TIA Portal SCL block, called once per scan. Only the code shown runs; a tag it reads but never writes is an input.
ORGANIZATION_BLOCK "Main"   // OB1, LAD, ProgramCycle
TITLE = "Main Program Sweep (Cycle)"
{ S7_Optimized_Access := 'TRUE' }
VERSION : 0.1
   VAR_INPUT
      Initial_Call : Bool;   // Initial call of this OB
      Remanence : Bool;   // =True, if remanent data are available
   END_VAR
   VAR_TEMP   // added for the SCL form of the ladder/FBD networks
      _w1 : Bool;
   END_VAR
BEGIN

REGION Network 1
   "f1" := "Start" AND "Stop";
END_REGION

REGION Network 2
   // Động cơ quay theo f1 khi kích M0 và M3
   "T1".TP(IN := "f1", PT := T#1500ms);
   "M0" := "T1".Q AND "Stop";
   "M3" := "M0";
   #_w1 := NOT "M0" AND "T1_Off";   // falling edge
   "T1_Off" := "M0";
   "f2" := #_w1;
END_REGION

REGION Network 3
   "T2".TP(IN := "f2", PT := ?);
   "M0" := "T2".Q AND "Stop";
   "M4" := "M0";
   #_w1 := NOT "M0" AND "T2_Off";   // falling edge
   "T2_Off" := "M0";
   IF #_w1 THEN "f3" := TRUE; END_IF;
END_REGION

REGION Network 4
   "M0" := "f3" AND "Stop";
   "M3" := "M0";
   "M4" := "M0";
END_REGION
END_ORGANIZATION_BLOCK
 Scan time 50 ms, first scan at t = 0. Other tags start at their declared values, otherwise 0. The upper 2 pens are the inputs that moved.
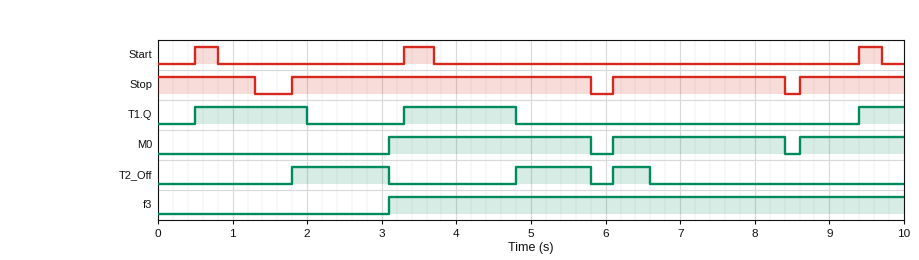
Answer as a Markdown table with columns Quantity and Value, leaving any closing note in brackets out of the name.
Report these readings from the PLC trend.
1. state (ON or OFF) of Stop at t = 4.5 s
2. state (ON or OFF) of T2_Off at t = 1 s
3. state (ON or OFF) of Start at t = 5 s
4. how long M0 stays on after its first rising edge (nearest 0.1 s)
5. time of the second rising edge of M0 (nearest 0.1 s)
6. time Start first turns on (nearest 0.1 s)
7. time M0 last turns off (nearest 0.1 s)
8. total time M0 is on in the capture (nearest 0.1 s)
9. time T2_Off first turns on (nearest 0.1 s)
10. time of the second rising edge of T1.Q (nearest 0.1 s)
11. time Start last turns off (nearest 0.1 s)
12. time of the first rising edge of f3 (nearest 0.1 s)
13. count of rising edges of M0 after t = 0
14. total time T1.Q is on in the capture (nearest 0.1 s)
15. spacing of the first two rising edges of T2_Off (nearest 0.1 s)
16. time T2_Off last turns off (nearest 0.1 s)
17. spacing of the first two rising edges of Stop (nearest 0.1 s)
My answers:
| Quantity | Value |
|---|---|
| state (ON or OFF) of Stop at t = 4.5 s | ON |
| state (ON or OFF) of T2_Off at t = 1 s | OFF |
| state (ON or OFF) of Start at t = 5 s | OFF |
| how long M0 stays on after its first rising edge | 2.7 s |
| time of the second rising edge of M0 | 6.1 s |
| time Start first turns on | 0.5 s |
| time M0 last turns off | 8.4 s |
| total time M0 is on in the capture | 6.4 s |
| time T2_Off first turns on | 1.8 s |
| time of the second rising edge of T1.Q | 3.3 s |
| time Start last turns off | 9.7 s |
| time of the first rising edge of f3 | 3.1 s |
| count of rising edges of M0 after t = 0 | 3 |
| total time T1.Q is on in the capture | 3.6 s |
| spacing of the first two rising edges of T2_Off | 3.0 s |
| time T2_Off last turns off | 6.6 s |
| spacing of the first two rising edges of Stop | 4.3 s |
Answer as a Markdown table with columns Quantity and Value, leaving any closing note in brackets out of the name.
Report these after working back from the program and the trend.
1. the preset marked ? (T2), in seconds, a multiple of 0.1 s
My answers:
| Quantity | Value |
|---|---|
| the preset marked ? (T2), in seconds, a multiple of 0.1 s | 1.8 s |
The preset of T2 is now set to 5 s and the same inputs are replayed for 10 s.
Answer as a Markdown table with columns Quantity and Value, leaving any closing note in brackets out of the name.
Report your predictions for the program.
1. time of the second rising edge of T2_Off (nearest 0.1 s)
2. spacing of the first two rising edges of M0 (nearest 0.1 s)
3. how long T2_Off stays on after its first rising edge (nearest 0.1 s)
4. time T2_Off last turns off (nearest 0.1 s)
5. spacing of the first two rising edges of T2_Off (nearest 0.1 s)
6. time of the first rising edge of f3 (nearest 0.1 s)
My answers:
| Quantity | Value |
|---|---|
| time of the second rising edge of T2_Off | 6.1 s |
| spacing of the first two rising edges of M0 | 2.5 s |
| how long T2_Off stays on after its first rising edge | 4.0 s |
| time T2_Off last turns off | 6.3 s |
| spacing of the first two rising edges of T2_Off | 4.3 s |
| time of the first rising edge of f3 | 5.8 s |
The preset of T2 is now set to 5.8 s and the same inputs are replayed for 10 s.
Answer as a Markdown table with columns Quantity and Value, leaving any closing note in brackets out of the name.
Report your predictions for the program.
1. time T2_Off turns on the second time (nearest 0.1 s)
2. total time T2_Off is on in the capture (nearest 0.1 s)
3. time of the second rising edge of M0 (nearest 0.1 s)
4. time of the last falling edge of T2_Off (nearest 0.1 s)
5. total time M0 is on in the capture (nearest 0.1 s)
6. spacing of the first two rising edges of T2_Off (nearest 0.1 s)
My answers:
| Quantity | Value |
|---|---|
| time T2_Off turns on the second time | 6.1 s |
| total time T2_Off is on in the capture | 5.0 s |
| time of the second rising edge of M0 | 8.6 s |
| time of the last falling edge of T2_Off | 7.1 s |
| total time M0 is on in the capture | 3.7 s |
| spacing of the first two rising edges of T2_Off | 4.3 s |
